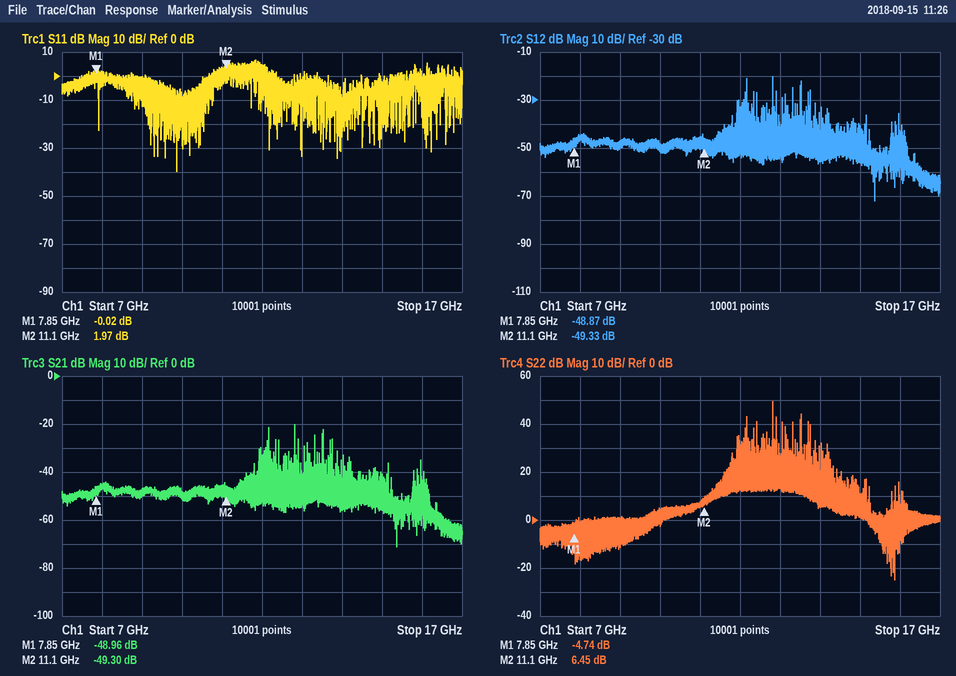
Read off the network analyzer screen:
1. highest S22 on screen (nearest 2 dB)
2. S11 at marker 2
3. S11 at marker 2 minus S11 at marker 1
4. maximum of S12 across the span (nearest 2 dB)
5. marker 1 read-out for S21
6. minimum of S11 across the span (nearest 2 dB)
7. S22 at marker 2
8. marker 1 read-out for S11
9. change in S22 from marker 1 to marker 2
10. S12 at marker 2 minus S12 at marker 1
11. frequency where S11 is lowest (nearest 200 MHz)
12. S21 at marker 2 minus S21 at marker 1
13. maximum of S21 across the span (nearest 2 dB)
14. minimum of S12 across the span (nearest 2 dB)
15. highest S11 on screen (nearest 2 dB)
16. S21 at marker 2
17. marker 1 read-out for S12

50 dB
1.97 dB
1.99 dB
-20 dB
-48.96 dB
-40 dB
6.45 dB
-0.02 dB
11.19 dB
-0.46 dB
9.8 GHz
-0.34 dB
-20 dB
-72 dB
6 dB
-49.30 dB
-48.87 dB
